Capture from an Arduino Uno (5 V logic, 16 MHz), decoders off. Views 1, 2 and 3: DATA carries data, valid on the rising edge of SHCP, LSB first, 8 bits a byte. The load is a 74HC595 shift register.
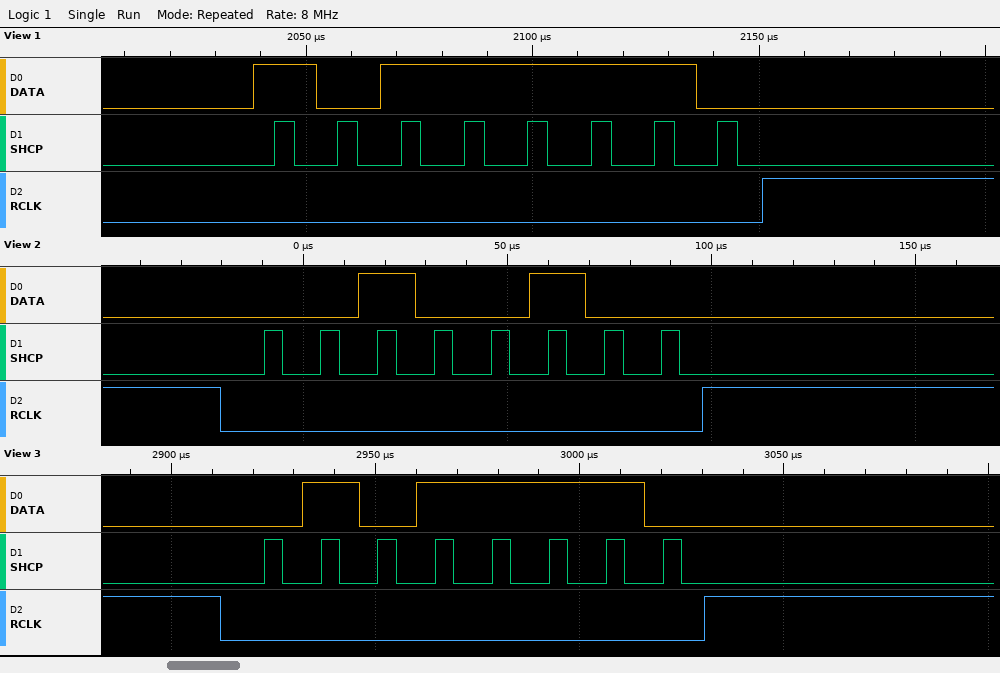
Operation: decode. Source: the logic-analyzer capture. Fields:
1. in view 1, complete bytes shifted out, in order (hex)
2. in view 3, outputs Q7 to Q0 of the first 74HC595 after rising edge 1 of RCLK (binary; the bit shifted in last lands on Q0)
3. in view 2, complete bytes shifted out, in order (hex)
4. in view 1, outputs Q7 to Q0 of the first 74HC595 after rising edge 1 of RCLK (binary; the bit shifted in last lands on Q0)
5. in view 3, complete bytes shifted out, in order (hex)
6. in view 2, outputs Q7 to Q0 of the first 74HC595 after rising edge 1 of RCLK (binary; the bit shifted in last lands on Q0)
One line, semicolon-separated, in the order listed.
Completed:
7D; 01011110; 24; 10111110; 7A; 00100100
